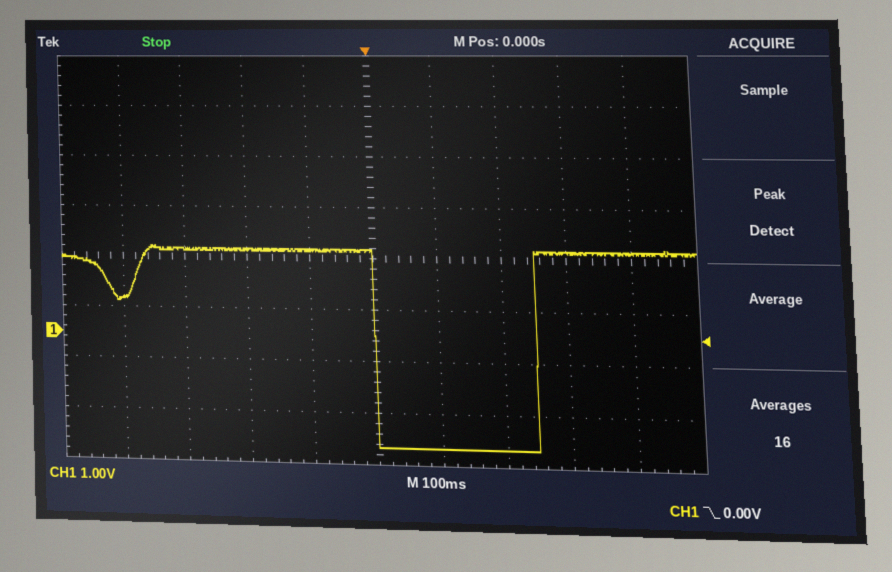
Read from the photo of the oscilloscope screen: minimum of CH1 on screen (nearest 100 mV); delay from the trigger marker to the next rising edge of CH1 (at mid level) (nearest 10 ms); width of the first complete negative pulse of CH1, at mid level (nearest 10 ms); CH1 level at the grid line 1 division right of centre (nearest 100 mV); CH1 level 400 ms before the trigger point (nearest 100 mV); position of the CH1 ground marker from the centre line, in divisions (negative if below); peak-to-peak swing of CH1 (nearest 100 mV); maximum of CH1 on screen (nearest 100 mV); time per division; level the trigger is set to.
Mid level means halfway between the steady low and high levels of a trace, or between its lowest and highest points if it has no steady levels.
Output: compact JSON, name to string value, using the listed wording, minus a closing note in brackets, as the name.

{"minimum of CH1 on screen": "-2.2 V", "delay from the trigger marker to the next rising edge of CH1 (at mid level)": "250 ms", "width of the first complete negative pulse of CH1, at mid level": "250 ms", "CH1 level at the grid line 1 division right of centre": "-2.2 V", "CH1 level 400 ms before the trigger point": "700 mV", "position of the CH1 ground marker from the centre line, in divisions": "-1.5 div", "peak-to-peak swing of CH1": "3.9 V", "maximum of CH1 on screen": "1.7 V", "time per division": "100 ms", "level the trigger is set to": "0.00 V"}
